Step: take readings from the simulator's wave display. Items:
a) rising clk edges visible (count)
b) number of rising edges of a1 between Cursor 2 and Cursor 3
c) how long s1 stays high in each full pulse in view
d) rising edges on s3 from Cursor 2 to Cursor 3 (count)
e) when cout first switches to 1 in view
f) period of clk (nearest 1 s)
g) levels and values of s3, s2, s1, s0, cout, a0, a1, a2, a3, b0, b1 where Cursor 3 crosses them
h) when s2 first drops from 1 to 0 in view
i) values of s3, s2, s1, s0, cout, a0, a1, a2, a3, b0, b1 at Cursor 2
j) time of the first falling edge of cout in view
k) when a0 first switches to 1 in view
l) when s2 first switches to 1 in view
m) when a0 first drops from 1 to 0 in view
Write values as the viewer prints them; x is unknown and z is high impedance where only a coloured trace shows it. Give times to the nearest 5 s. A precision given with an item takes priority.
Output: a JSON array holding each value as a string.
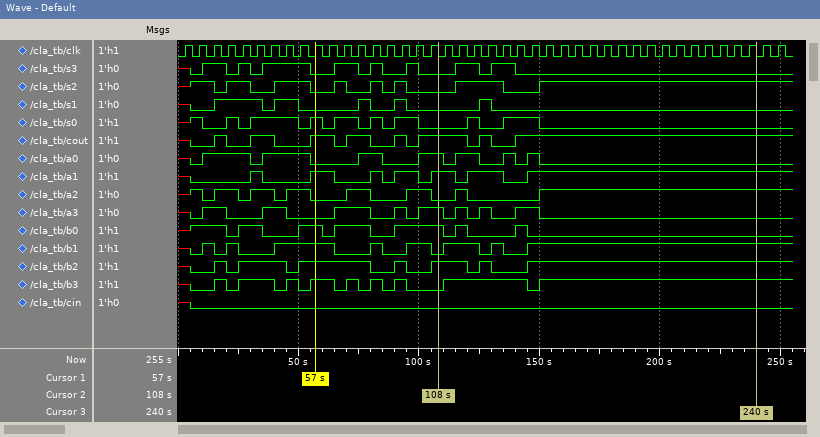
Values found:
["42", "2", "20 s, 10 s, 5 s, 5 s, 5 s", "2", "15 s", "6 s", "s3=0, s2=1, s1=0, s0=0, cout=1, a0=0, a1=1, a2=1, a3=0, b0=0, b1=1", "15 s", "s3=0, s2=0, s1=0, s0=0, cout=1, a0=1, a1=1, a2=0, a3=1, b0=1, b1=0", "20 s", "10 s", "5 s", "30 s"]
